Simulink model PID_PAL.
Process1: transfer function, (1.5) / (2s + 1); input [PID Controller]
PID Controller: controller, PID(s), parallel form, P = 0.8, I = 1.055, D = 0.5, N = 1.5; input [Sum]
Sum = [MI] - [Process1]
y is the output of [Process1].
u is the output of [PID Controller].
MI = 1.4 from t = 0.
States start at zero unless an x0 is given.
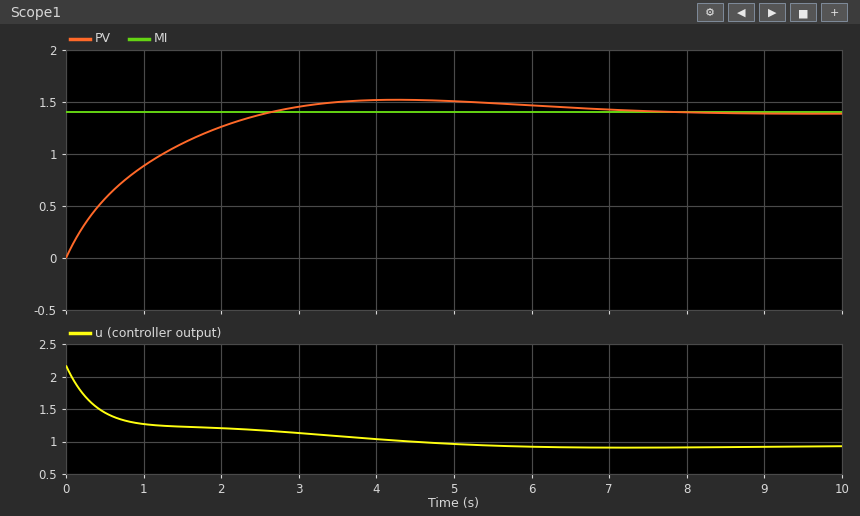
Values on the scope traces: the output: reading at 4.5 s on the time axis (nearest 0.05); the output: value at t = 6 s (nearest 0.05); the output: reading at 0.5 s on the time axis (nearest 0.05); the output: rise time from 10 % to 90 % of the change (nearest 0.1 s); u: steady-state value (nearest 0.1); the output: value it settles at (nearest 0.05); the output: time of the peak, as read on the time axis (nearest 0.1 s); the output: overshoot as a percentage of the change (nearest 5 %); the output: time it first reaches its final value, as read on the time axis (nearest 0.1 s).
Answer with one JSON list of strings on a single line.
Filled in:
["1.50", "1.45", "0.55", "1.9 s", "0.9", "1.40", "4.3 s", "10 %", "2.6 s"]
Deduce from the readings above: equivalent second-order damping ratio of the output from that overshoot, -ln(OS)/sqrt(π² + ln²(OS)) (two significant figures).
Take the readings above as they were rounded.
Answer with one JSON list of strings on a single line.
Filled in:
["0.59"]
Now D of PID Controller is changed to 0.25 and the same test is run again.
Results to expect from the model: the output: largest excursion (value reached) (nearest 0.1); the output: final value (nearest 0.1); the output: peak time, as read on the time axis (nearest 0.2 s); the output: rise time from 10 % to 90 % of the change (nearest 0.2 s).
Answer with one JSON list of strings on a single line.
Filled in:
["1.5", "1.4", "3.8 s", "1.8 s"]
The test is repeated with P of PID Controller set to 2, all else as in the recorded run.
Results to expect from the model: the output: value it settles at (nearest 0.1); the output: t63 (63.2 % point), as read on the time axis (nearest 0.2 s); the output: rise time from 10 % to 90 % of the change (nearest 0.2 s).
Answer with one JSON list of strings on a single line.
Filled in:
["1.4", "0.6 s", "1.6 s"]
